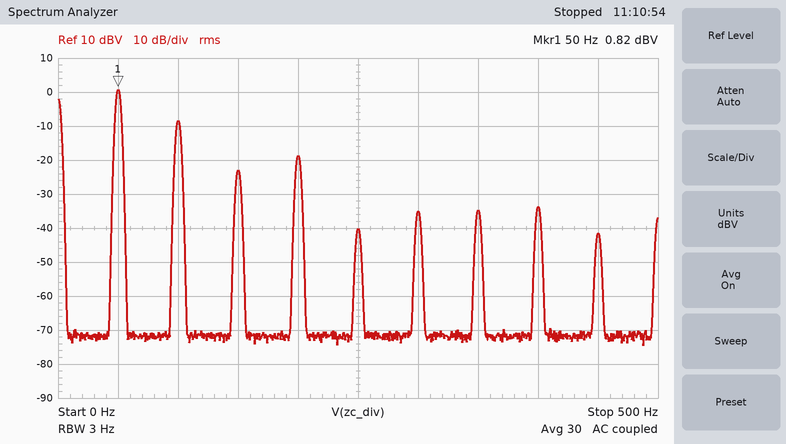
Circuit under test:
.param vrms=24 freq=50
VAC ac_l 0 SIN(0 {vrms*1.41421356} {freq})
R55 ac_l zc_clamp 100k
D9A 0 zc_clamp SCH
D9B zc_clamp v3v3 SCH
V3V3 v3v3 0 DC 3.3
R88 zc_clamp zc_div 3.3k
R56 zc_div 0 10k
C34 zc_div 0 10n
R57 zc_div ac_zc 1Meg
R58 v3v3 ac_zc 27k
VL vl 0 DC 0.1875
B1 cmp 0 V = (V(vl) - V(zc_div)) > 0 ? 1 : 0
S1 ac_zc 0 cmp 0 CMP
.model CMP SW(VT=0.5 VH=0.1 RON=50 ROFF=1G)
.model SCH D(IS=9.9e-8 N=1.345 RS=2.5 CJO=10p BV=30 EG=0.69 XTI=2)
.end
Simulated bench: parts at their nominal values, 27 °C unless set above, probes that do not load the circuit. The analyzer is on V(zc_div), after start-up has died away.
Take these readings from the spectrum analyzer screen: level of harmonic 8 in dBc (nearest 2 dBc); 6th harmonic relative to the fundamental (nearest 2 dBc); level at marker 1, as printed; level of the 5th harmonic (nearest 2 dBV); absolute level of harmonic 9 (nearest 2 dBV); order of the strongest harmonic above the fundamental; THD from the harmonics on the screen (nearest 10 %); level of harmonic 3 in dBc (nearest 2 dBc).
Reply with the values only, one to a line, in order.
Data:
-34 dBc
-36 dBc
0.82 dBV
-40 dBV
-42 dBV
2
40 %
-24 dBc
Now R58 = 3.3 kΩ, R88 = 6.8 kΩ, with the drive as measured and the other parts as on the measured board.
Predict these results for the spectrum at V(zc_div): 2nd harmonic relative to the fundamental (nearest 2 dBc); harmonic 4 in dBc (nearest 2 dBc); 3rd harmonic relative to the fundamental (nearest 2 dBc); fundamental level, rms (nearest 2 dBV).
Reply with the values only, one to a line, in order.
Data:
-10 dBc
-16 dBc
-18 dBc
0 dBV
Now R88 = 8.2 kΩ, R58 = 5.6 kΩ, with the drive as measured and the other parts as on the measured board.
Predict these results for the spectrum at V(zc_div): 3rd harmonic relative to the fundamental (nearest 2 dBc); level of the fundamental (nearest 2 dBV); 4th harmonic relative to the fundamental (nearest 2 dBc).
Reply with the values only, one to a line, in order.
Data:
-16 dBc
-2 dBV
-16 dBc
